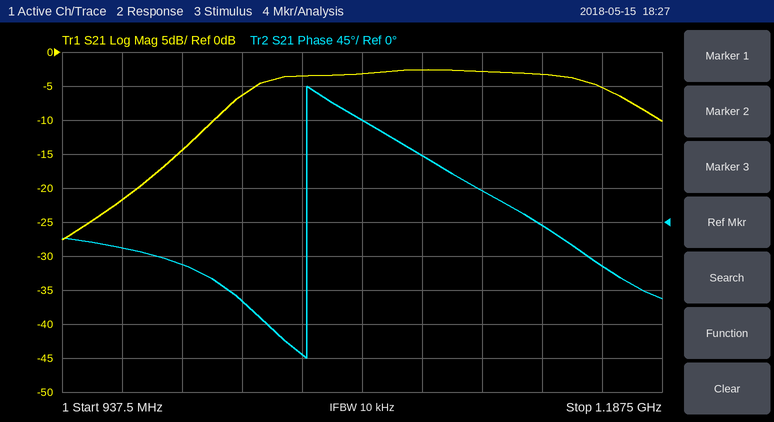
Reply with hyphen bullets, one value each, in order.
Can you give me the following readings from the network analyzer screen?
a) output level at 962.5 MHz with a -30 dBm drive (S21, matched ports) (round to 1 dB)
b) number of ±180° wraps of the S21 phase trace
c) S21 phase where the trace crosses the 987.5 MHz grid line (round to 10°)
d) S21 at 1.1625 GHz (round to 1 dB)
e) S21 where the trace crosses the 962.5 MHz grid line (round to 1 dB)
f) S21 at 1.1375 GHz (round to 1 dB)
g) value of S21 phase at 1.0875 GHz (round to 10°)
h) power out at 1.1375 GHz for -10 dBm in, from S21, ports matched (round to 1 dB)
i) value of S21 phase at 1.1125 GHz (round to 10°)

- -52 dBm
- 1
- -60°
- -5 dB
- -22 dB
- -3 dB
- 90°
- -13 dBm
- 40°
